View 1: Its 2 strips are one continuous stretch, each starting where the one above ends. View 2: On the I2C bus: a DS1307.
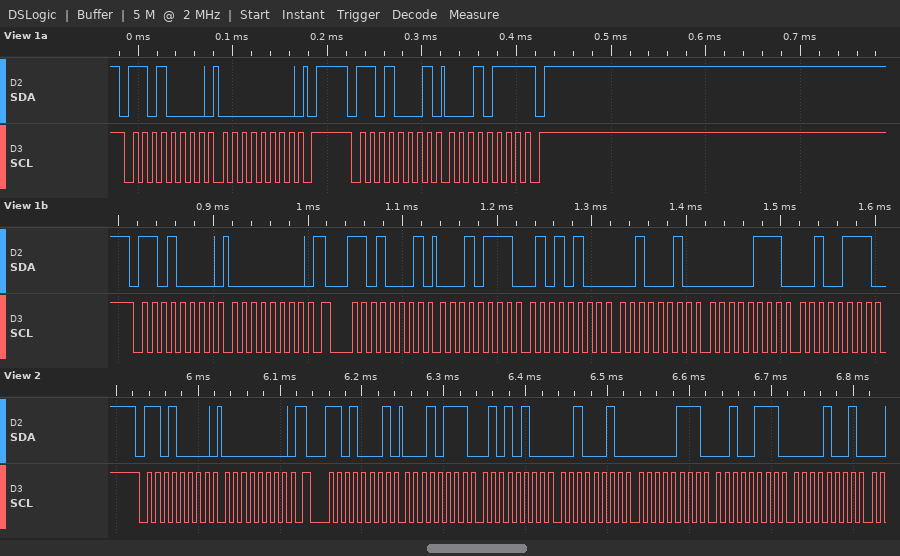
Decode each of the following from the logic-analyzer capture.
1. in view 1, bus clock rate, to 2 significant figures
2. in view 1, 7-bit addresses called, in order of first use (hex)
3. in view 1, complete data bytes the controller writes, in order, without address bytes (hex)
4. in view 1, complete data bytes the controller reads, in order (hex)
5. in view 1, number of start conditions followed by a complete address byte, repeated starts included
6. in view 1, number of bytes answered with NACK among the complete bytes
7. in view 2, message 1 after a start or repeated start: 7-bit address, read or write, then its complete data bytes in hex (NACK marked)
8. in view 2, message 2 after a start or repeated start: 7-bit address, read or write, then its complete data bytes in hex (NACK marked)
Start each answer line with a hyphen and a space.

- 100 kHz
- 0x68
- 00 00
- 17 17 54 22 07 27
- 4
- 1
- 0x68 write: 00
- 0x68 read: 17 54 22 07 27 09
